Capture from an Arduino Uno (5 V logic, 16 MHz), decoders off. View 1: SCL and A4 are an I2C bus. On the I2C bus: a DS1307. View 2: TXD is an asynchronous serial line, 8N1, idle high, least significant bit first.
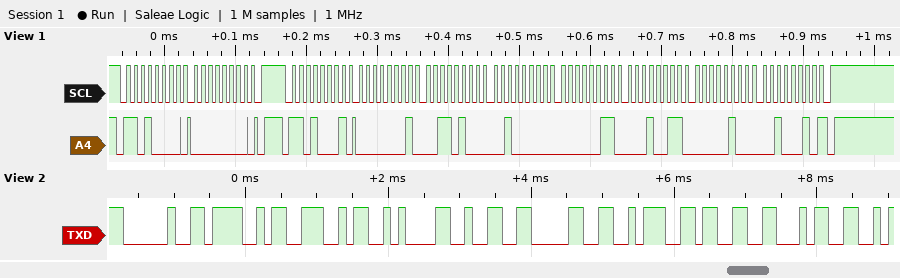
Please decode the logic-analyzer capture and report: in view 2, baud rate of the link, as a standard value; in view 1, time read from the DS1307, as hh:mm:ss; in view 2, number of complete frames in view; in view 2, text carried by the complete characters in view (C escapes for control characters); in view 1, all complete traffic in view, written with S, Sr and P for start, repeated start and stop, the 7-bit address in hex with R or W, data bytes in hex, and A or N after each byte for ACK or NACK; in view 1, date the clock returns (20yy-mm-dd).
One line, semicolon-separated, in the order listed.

9600 baud; 20:34:01; 9; " ON\n20:34"; S 68W A 00 A P S 68R A 01 A 34 A 20 A 03 A 13 A 04 A 22 N P; 2022-04-13
